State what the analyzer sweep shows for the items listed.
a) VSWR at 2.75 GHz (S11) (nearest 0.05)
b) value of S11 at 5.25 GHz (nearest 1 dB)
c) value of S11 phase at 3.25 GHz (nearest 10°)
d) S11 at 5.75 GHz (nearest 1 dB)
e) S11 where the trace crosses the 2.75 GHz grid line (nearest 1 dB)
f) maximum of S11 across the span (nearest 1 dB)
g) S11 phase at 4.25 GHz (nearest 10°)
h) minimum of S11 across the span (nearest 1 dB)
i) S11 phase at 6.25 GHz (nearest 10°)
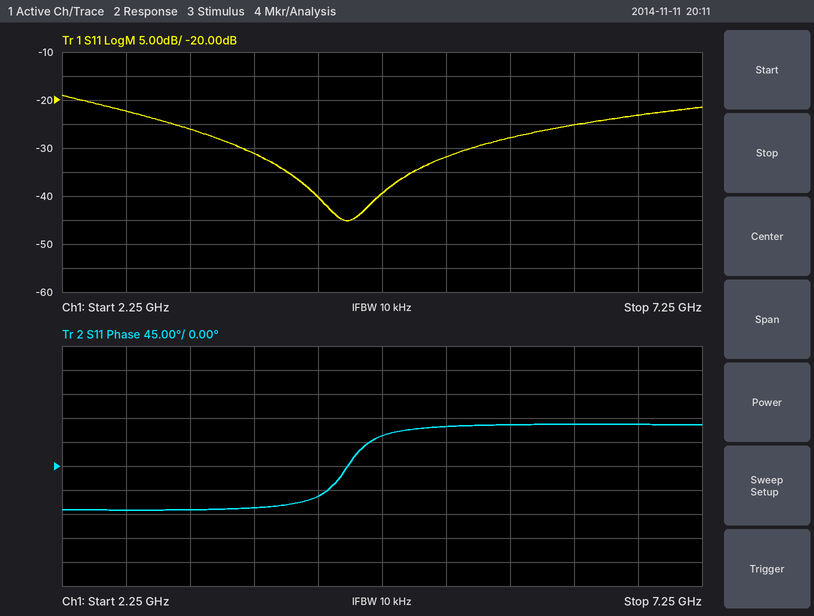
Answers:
1.15
-32 dB
-80°
-28 dB
-22 dB
-19 dB
-60°
-45 dB
80°
